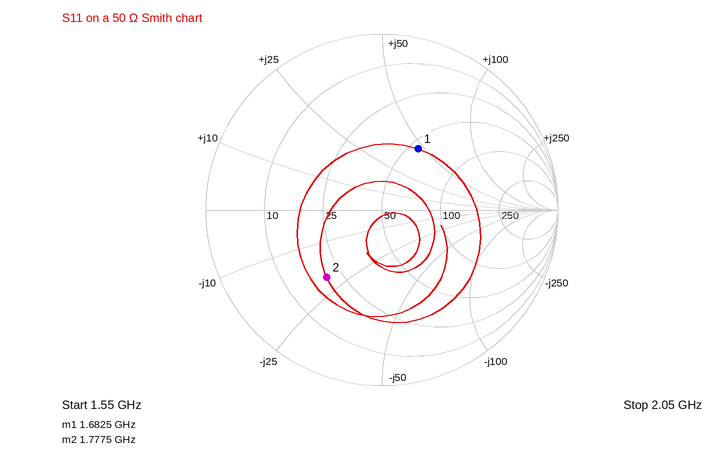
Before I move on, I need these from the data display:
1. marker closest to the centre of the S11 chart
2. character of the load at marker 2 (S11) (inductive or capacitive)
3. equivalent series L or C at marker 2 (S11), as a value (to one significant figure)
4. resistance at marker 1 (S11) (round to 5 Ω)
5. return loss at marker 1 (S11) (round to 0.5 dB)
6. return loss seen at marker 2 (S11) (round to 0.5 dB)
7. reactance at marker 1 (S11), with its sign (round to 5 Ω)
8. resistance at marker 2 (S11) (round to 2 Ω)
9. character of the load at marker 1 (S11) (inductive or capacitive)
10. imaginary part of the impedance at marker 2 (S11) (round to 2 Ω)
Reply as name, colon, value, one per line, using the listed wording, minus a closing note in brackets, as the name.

marker closest to the centre of the S11 chart: marker 1
character of the load at marker 2 (S11): capacitive
equivalent series L or C at marker 2 (S11), as a value: 4 pF
resistance at marker 1 (S11): 55 Ω
return loss at marker 1 (S11): 8.0 dB
return loss seen at marker 2 (S11): 6.0 dB
reactance at marker 1 (S11), with its sign: +45 Ω
resistance at marker 2 (S11): 20 Ω
character of the load at marker 1 (S11): inductive
imaginary part of the impedance at marker 2 (S11): -20 Ω
